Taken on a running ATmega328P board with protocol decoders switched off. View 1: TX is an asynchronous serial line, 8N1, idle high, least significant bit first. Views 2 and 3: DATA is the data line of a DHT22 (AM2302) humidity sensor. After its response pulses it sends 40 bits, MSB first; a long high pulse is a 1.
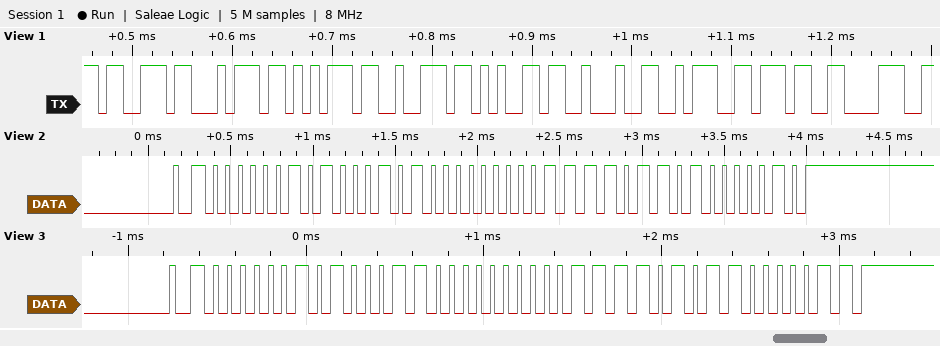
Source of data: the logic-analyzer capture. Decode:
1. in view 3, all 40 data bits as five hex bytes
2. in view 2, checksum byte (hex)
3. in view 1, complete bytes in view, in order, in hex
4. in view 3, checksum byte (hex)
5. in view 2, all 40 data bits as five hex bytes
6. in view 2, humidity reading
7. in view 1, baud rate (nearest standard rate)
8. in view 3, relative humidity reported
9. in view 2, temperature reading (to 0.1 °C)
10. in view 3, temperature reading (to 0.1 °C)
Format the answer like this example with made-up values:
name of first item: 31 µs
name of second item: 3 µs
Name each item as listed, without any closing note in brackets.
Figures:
in view 3, all 40 data bits as five hex bytes: 02 8C 00 F5 83
in view 2, checksum byte: 0x82
in view 1, complete bytes in view, in order, in hex: 73 74 75 72 65 22 3A 37 38
in view 3, checksum byte: 0x83
in view 2, all 40 data bits as five hex bytes: 02 8A 00 F6 82
in view 2, humidity reading: 65.0 %
in view 1, baud rate: 115200 baud
in view 3, relative humidity reported: 65.2 %
in view 2, temperature reading: 24.6 °C
in view 3, temperature reading: 24.5 °C
